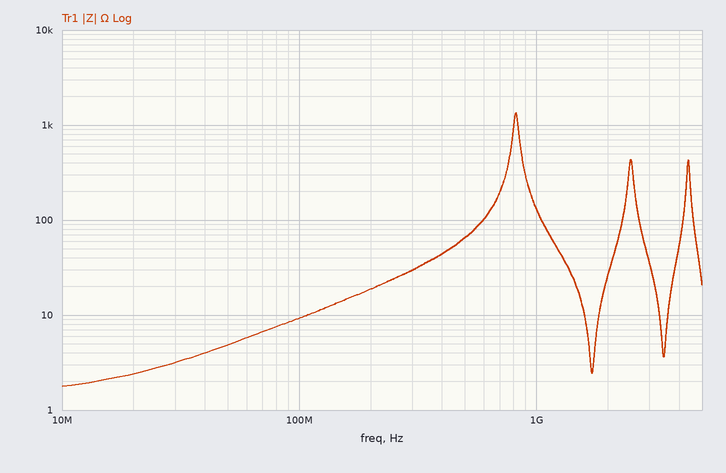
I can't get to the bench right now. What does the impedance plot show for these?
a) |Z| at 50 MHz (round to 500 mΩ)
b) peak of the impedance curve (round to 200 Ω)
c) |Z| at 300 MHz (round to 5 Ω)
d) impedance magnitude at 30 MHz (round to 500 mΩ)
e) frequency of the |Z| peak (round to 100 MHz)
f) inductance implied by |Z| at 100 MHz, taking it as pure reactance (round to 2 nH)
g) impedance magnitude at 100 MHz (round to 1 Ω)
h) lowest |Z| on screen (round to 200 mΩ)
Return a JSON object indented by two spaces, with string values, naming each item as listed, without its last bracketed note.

{
  "|Z| at 50 MHz": "5.0 Ω",
  "peak of the impedance curve": "1.4 kΩ",
  "|Z| at 300 MHz": "30 Ω",
  "impedance magnitude at 30 MHz": "3.0 Ω",
  "frequency of the |Z| peak": "800 MHz",
  "inductance implied by |Z| at 100 MHz, taking it as pure reactance": "14 nH",
  "impedance magnitude at 100 MHz": "9 Ω",
  "lowest |Z| on screen": "1.8 Ω"
}
